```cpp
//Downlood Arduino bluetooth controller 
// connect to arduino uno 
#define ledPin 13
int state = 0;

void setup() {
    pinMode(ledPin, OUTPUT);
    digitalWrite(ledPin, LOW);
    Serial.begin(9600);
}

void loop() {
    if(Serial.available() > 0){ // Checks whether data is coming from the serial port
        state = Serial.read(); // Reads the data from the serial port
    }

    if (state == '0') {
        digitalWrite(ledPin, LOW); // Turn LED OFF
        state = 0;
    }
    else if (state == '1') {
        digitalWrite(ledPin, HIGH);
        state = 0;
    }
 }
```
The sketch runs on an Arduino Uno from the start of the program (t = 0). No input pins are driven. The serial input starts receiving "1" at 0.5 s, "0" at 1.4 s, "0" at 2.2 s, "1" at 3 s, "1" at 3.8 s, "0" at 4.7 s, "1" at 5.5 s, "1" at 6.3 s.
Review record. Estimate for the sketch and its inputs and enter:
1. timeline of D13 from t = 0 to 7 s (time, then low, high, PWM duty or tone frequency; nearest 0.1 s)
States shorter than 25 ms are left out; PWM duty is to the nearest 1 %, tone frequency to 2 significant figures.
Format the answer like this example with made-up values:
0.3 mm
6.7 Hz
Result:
0 s low; 0.5 s high; 1.4 s low; 3 s high; 4.7 s low; 5.5 s high
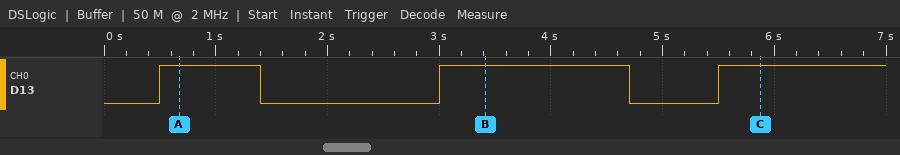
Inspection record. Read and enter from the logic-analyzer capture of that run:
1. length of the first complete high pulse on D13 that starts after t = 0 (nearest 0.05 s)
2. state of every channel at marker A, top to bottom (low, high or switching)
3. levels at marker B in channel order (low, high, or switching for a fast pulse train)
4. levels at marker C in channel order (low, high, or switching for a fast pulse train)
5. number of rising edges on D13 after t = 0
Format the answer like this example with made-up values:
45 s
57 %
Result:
0.90 s
D13 high
D13 high
D13 high
3
